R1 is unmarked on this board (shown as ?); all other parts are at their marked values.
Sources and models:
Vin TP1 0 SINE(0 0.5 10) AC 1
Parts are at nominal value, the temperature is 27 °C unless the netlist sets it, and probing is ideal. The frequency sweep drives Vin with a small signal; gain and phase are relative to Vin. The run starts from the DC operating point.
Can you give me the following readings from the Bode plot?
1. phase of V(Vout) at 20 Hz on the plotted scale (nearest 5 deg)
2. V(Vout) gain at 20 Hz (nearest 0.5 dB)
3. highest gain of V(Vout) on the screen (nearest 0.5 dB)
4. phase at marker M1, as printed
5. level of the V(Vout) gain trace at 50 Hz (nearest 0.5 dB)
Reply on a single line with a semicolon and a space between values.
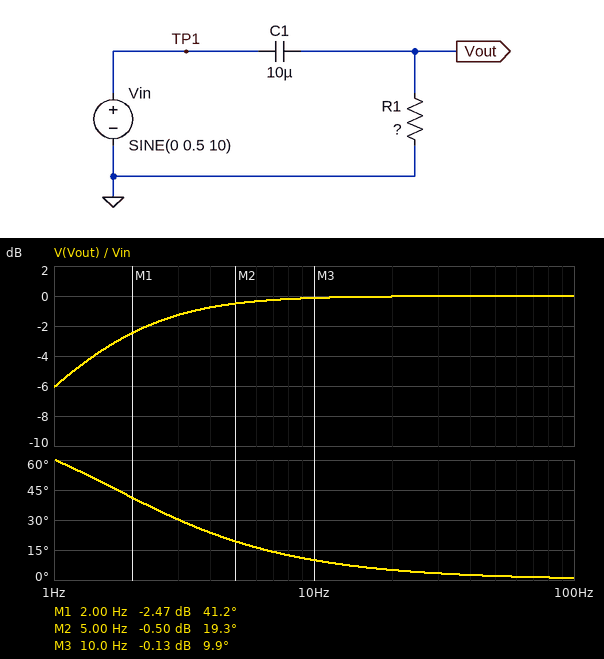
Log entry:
5 deg; 0 dB; 0 dB; 41.2 deg; 0 dB
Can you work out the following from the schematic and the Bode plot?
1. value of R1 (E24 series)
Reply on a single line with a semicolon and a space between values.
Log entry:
9.1 kΩ
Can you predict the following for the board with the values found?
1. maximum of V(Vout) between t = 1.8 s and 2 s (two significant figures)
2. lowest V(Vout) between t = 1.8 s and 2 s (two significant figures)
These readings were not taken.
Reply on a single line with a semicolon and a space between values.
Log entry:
490 mV; -490 mV
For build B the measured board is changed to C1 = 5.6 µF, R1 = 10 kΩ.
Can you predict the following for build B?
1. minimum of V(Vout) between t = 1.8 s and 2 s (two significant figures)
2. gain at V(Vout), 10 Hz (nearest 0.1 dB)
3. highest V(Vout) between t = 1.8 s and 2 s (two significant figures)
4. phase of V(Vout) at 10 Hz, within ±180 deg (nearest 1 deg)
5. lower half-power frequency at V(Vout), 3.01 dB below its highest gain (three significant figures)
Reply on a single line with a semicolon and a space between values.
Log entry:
-480 mV; -0.3 dB; 480 mV; 16 deg; 2.84 Hz
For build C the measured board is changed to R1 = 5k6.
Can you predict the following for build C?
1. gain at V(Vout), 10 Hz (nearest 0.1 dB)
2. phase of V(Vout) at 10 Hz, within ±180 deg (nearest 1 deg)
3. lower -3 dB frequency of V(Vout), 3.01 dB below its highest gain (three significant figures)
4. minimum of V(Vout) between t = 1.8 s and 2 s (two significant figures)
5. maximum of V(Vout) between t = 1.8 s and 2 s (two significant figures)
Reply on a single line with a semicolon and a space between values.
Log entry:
-0.3 dB; 16 deg; 2.84 Hz; -480 mV; 480 mV
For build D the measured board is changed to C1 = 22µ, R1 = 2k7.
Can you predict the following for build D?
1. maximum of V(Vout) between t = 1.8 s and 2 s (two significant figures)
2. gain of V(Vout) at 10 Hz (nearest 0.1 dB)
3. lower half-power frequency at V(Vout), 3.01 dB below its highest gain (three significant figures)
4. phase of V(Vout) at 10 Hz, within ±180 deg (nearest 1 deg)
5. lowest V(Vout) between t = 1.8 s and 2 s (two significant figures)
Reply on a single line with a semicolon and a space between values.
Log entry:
480 mV; -0.3 dB; 2.68 Hz; 15 deg; -480 mV
